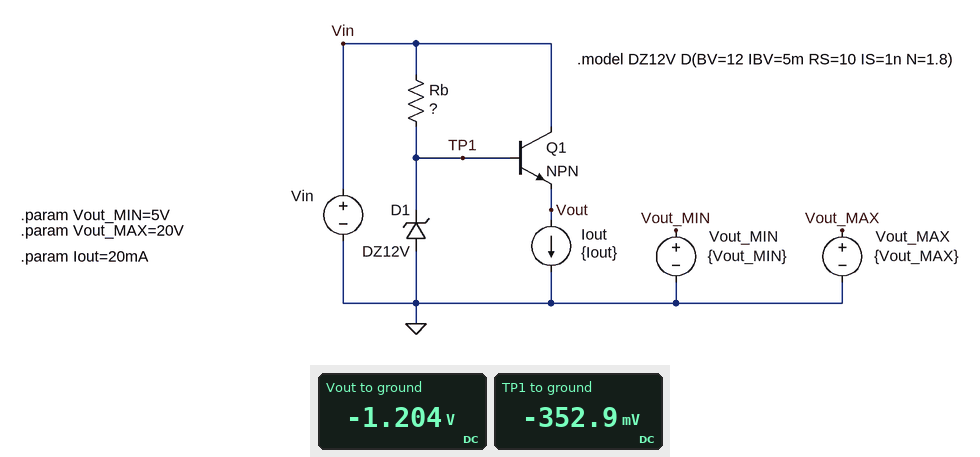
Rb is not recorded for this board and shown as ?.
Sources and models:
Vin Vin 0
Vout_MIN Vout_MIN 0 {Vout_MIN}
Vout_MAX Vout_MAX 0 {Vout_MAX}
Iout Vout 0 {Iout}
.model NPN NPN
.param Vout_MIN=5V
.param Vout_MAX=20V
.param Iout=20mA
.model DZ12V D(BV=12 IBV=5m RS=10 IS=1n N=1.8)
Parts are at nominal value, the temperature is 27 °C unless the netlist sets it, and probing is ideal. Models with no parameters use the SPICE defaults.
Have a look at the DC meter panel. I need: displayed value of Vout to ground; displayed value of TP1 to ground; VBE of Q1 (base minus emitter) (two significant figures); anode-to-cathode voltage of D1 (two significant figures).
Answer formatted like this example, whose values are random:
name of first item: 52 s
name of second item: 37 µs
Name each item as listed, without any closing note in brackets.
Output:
displayed value of Vout to ground: -1.204 V
displayed value of TP1 to ground: -352.9 mV
VBE of Q1 (base minus emitter): 850 mV
anode-to-cathode voltage of D1: 350 mV
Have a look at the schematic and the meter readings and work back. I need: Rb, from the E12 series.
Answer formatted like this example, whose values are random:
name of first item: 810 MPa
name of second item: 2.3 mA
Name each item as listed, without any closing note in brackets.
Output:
Rb, from the E12 series: 1.8 kΩ
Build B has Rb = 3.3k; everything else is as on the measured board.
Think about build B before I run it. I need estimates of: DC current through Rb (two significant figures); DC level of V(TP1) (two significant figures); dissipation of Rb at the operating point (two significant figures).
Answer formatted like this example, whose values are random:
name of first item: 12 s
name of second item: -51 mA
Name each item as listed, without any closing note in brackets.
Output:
DC current through Rb: 150 µA
DC level of V(TP1): -500 mV
dissipation of Rb at the operating point: 76 µW
